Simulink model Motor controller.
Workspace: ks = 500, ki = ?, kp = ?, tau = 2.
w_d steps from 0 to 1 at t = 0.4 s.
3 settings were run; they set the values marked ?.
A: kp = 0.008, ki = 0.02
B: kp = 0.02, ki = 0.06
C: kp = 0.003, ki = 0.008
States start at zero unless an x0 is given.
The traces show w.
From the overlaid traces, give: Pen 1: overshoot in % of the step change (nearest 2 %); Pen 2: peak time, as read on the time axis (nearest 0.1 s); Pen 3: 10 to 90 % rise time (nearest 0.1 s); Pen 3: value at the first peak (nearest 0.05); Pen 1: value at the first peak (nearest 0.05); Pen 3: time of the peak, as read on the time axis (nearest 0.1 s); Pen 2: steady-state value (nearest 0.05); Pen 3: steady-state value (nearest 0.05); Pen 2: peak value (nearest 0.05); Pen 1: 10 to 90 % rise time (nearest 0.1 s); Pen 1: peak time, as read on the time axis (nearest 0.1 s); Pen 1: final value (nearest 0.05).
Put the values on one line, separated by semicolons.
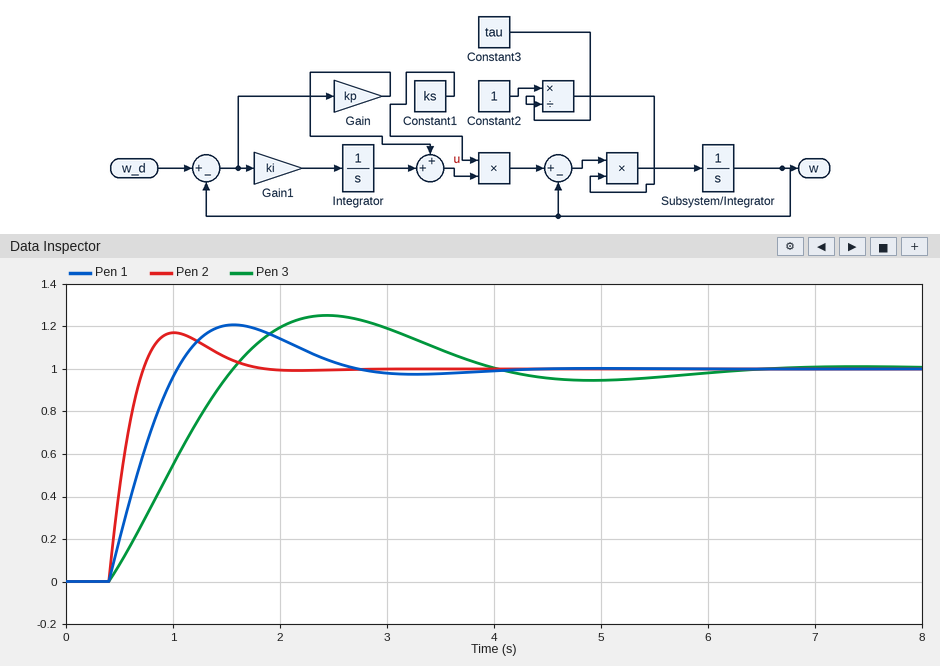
20 %; 1.0 s; 0.9 s; 1.25; 1.20; 2.4 s; 1.00; 1.00; 1.15; 0.5 s; 1.6 s; 1.00
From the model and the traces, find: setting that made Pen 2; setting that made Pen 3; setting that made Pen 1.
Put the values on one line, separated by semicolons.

B; C; A
